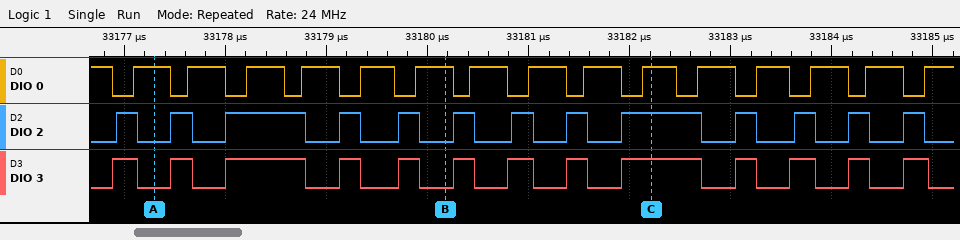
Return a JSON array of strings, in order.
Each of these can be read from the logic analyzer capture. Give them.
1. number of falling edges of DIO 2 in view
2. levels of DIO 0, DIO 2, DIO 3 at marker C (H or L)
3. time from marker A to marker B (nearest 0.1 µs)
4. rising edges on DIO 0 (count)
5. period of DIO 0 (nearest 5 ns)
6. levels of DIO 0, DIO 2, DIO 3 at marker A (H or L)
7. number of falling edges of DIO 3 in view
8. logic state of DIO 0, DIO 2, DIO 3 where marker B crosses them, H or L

["13", "DIO 0=H, DIO 2=H, DIO 3=H", "2.9 µs", "15", "560 ns", "DIO 0=H, DIO 2=L, DIO 3=L", "13", "DIO 0=H, DIO 2=L, DIO 3=L"]
